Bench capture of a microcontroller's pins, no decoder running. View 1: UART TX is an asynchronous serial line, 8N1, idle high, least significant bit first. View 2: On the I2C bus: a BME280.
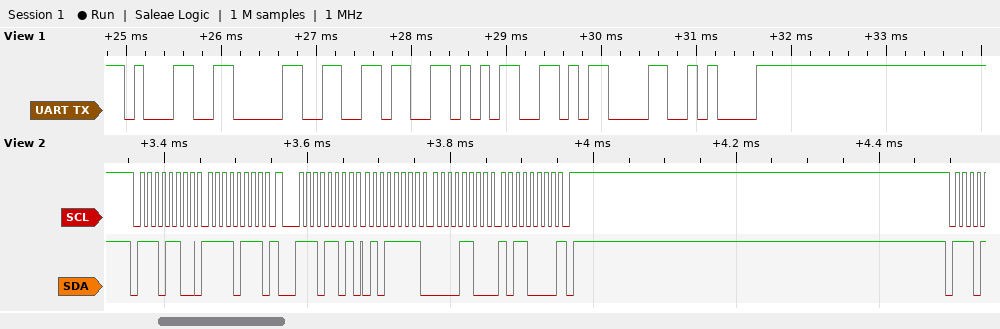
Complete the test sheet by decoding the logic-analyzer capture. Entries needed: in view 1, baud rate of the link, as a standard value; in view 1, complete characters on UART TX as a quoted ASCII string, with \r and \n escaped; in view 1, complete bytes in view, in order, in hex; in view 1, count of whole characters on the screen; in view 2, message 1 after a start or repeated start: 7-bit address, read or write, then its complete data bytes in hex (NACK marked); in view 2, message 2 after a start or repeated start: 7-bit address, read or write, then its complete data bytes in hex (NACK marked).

9600 baud
"1065\r\n"
31 30 36 35 0D 0A
6
0x76 write: F7
0x76 read: 5F 0C B0 NACK
